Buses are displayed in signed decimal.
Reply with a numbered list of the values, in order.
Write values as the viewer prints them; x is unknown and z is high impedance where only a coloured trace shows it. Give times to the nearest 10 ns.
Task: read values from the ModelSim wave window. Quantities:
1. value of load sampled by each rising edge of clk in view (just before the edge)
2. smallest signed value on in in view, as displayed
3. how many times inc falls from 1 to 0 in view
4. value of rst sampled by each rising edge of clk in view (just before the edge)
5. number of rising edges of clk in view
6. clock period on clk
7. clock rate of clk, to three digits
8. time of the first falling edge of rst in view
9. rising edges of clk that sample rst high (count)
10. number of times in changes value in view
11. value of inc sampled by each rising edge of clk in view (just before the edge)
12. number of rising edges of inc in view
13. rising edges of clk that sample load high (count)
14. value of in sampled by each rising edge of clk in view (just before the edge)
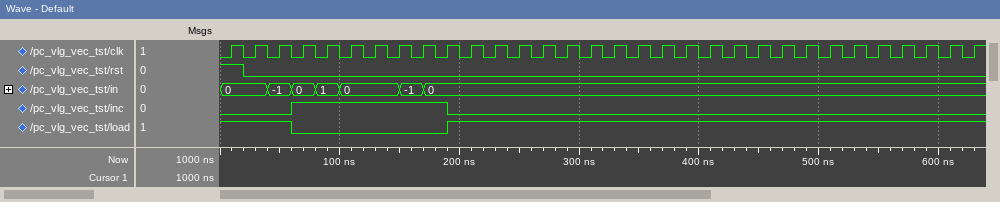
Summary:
1. 1 1 1 0 0 0 0 0 0 0 1 1 1 1 1 1 1 1 1 1 1 1 1 1 1 1 1 1 1 1 1 1
2. -1
3. 1
4. 1 0 0 0 0 0 0 0 0 0 0 0 0 0 0 0 0 0 0 0 0 0 0 0 0 0 0 0 0 0 0 0
5. 32
6. 20 ns
7. 50.0 MHz
8. 20 ns
9. 1
10. 6
11. 0 0 0 1 1 1 1 1 1 1 0 0 0 0 0 0 0 0 0 0 0 0 0 0 0 0 0 0 0 0 0 0
12. 1
13. 25
14. 0, 0, -1, 0, 1, 0, 0, 0, -1, 0, 0, 0, 0, 0, 0, 0, 0, 0, 0, 0, 0, 0, 0, 0, 0, 0, 0, 0, 0, 0, 0, 0
